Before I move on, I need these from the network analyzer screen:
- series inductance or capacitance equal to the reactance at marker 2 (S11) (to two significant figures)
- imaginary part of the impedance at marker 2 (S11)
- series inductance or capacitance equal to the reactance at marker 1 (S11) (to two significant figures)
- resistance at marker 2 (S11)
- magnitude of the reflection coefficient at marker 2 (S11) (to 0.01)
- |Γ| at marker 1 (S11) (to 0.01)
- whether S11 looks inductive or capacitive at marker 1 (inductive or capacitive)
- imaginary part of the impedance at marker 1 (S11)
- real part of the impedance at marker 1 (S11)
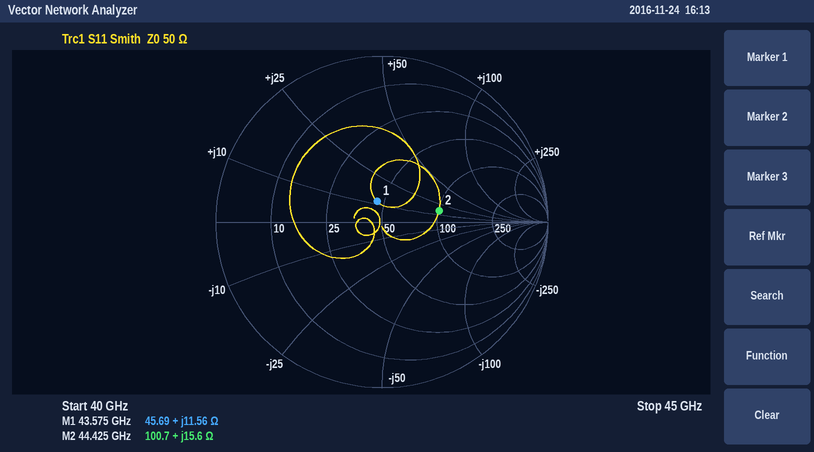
56 pH
+15.6 Ω
42 pH
100.7 Ω
0.35
0.13
inductive
+11.56 Ω
45.69 Ω
